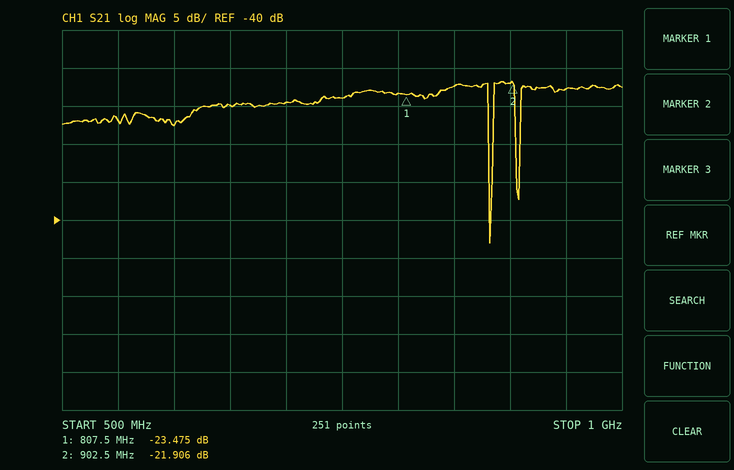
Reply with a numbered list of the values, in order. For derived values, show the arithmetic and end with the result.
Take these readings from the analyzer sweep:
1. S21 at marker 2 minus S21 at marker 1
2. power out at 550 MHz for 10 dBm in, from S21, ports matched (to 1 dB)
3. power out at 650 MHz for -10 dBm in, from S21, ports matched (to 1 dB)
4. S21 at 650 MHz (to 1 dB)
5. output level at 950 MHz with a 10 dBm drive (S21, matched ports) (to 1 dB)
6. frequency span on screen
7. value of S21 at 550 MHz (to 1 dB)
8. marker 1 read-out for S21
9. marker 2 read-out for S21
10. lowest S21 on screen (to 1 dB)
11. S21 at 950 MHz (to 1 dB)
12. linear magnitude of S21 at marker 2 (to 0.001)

1. -21.906 − (-23.475) = 1.569 dB
2. 10 dBm + (-27 dB) = -17 dBm
3. -10 dBm + (-25 dB) = -35 dBm
4. -25 dB
5. 10 dBm + (-23 dB) = -13 dBm
6. 500 MHz
7. -27 dB
8. -23.475 dB
9. -21.906 dB
10. -43 dB
11. -23 dB
12. 10^(-21.906/20) ≈ 0.080
